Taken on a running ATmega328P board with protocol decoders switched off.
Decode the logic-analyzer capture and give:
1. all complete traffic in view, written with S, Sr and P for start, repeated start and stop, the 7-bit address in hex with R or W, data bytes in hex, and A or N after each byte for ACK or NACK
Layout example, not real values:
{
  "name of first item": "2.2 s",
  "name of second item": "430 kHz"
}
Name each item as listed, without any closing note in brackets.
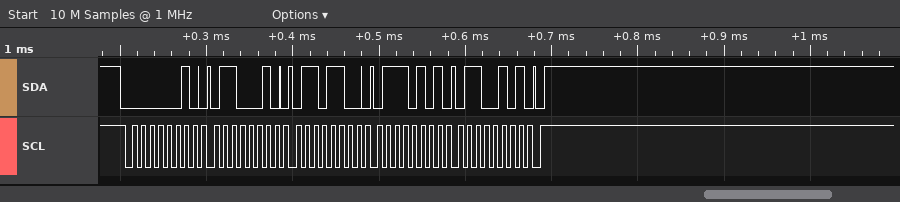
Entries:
{
  "all complete traffic in view, written with S, Sr and P for start, repeated start and stop, the 7-bit address in hex with R or W, data bytes in hex, and A or N after each byte for ACK or NACK": "S 01W A 62 A 6C A 75 A 65 A P"
}
